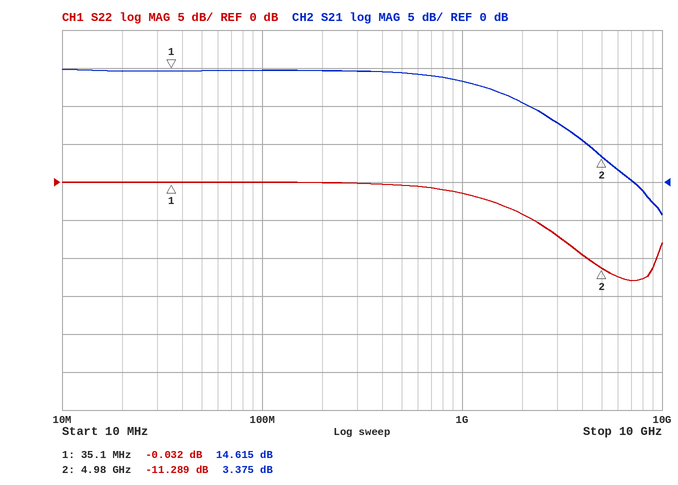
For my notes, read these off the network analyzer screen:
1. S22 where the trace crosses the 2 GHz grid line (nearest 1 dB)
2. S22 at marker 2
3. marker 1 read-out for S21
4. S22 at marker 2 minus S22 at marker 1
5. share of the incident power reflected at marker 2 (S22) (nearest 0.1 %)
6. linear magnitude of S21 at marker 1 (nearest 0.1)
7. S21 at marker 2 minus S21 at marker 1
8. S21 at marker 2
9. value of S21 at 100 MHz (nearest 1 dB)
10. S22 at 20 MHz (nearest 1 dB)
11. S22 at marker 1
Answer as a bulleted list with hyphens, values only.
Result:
- -4 dB
- -11.289 dB
- 14.615 dB
- -11.257 dB
- 7.4 %
- 5.4
- -11.240 dB
- 3.375 dB
- 15 dB
- 0 dB
- -0.032 dB
